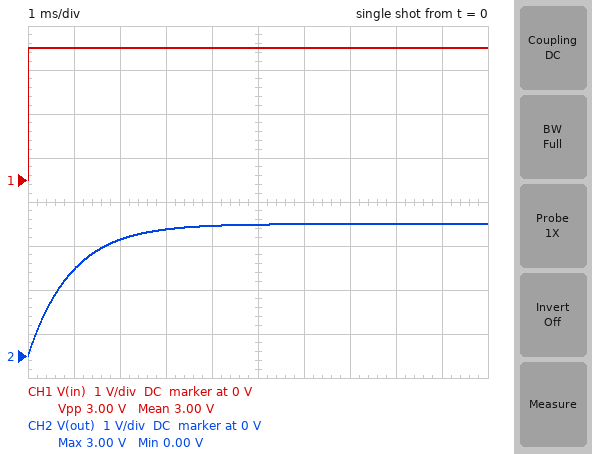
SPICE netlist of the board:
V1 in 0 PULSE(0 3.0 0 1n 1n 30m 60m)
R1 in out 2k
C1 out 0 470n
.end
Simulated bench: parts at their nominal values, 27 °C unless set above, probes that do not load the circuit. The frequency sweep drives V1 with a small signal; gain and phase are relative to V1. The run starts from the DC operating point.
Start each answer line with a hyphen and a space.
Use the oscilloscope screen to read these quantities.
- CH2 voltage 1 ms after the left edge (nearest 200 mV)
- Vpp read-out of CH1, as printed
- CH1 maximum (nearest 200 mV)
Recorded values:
- 2.0 V
- 3.00 V
- 3.0 V
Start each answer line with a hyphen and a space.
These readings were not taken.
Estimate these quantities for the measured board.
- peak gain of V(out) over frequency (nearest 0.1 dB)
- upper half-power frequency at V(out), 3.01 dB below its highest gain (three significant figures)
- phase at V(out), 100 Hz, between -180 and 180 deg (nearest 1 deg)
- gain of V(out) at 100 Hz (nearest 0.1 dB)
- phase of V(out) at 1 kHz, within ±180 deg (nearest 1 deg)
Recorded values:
- 0 dB
- 169 Hz
- -31 deg
- -1.3 dB
- -80 deg
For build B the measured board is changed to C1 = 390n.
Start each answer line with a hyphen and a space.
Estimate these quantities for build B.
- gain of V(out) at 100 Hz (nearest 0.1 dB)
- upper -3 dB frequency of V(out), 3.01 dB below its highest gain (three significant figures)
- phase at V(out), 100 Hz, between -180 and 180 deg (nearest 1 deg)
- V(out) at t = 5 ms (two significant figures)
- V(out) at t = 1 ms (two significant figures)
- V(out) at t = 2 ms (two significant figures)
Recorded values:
- -0.9 dB
- 204 Hz
- -26 deg
- 3.0 V
- 2.2 V
- 2.8 V
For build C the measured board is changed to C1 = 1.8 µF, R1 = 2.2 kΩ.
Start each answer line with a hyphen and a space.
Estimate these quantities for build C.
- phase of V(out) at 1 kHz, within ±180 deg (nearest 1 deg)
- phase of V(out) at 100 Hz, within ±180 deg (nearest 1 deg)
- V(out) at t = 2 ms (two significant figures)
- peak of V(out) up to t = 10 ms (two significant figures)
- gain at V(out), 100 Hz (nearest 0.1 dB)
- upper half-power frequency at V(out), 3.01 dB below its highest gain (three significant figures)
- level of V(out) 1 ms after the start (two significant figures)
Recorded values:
- -88 deg
- -68 deg
- 1.2 V
- 2.8 V
- -8.6 dB
- 40.2 Hz
- 670 mV
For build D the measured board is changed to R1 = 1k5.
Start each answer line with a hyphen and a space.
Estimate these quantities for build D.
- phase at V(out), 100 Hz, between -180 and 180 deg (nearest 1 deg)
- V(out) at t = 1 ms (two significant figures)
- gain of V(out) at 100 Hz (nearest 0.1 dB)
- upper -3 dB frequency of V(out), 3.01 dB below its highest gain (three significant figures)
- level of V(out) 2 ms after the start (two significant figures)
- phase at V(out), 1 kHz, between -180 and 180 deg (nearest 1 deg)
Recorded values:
- -24 deg
- 2.3 V
- -0.8 dB
- 226 Hz
- 2.8 V
- -77 deg
